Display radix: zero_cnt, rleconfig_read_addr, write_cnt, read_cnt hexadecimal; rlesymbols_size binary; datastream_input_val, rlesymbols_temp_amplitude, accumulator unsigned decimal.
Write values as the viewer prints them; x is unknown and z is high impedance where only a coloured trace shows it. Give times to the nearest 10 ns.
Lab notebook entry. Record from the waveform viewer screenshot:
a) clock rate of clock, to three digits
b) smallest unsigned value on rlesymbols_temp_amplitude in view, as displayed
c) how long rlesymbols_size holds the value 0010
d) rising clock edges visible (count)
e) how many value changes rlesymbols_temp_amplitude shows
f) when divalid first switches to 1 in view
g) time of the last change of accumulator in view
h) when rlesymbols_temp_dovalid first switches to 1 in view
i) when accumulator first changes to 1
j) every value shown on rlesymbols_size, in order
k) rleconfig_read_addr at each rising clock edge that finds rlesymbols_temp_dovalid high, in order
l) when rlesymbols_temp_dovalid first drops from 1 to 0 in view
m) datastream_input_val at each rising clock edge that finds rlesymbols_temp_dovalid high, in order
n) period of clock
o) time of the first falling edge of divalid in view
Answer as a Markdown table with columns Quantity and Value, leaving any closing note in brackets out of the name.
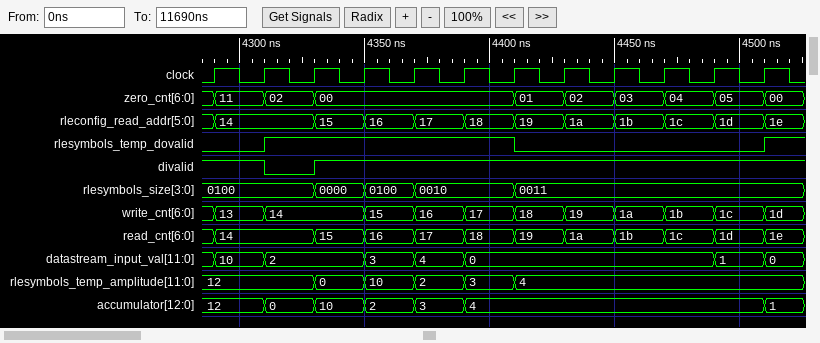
| Quantity | Value |
|---|---|
| clock rate of clock, to three digits | 50.0 MHz |
| smallest unsigned value on rlesymbols_temp_amplitude in view, as displayed | 0 |
| how long rlesymbols_size holds the value 0010 | 40 ns |
| rising clock edges visible | 12 |
| how many value changes rlesymbols_temp_amplitude shows | 5 |
| when divalid first switches to 1 in view | 4330 ns |
| time of the last change of accumulator in view | 4510 ns |
| when rlesymbols_temp_dovalid first switches to 1 in view | 4310 ns |
| when accumulator first changes to 1 | 4510 ns |
| every value shown on rlesymbols_size, in order | 0100, 0000, 0100, 0010, 0011 |
| rleconfig_read_addr at each rising clock edge that finds rlesymbols_temp_dovalid high, in order | 14, 15, 16, 17, 18 |
| when rlesymbols_temp_dovalid first drops from 1 to 0 in view | 4410 ns |
| datastream_input_val at each rising clock edge that finds rlesymbols_temp_dovalid high, in order | 2, 2, 3, 4, 0 |
| period of clock | 20 ns |
| time of the first falling edge of divalid in view | 4310 ns |
